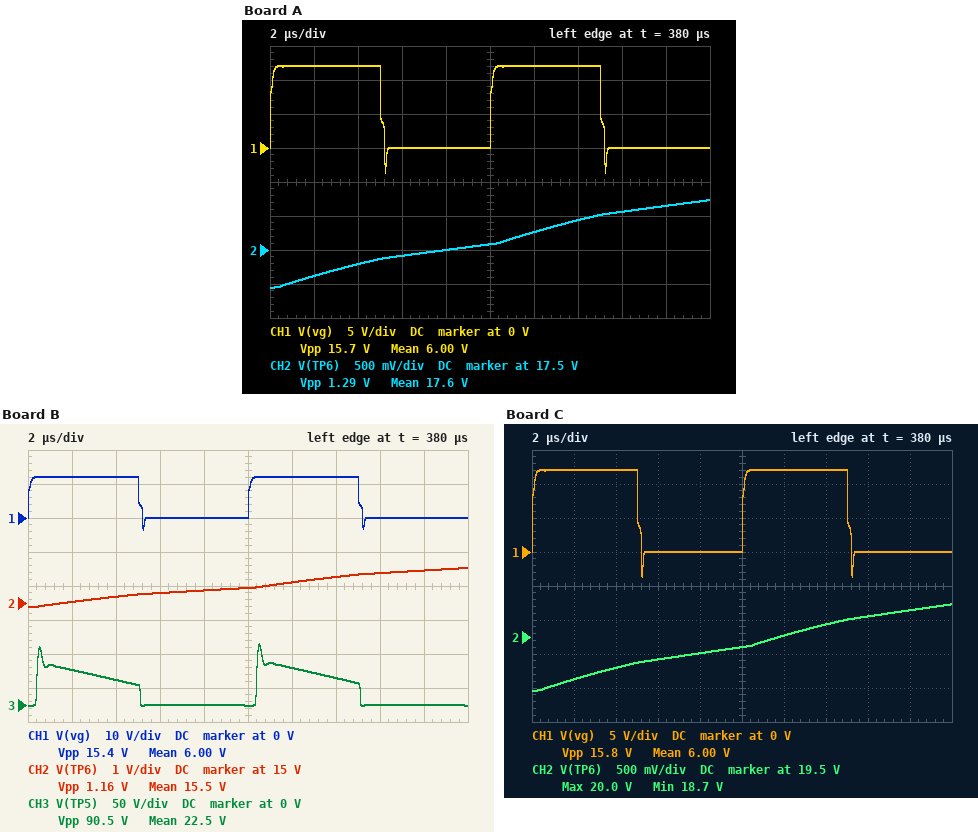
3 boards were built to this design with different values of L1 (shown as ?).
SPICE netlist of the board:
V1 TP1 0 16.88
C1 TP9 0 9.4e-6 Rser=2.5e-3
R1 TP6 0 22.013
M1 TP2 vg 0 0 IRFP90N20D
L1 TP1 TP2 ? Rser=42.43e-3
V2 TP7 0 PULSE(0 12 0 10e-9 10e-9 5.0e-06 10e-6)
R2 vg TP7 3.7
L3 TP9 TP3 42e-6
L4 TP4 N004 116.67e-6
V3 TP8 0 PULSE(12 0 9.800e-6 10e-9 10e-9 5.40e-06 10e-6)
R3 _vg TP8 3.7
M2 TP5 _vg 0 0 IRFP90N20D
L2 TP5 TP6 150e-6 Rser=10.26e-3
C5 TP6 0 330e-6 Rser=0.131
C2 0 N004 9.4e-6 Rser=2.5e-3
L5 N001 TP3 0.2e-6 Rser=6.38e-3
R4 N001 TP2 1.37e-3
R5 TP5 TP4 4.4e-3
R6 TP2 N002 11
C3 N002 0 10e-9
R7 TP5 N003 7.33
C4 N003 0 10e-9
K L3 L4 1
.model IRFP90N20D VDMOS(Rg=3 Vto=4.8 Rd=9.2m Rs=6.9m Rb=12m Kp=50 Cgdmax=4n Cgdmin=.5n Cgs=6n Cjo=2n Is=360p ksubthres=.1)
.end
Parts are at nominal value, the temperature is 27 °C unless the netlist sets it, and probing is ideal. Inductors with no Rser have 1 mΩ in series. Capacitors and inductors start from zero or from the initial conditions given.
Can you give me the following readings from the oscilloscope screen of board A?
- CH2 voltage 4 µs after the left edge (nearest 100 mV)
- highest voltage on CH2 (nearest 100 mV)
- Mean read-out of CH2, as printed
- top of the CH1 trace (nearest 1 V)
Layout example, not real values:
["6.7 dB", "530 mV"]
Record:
["17.3 V", "18.2 V", "17.6 V", "12 V"]
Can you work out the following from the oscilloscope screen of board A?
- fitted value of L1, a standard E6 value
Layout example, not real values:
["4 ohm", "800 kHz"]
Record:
["47 µH"]
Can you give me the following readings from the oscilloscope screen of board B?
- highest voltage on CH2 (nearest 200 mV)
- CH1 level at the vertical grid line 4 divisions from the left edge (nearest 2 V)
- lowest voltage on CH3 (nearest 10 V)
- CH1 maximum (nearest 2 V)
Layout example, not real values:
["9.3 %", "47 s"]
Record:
["16.0 V", "0 V", "0 V", "12 V"]
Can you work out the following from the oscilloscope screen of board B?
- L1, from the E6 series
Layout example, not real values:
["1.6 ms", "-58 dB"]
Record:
["68 µH"]
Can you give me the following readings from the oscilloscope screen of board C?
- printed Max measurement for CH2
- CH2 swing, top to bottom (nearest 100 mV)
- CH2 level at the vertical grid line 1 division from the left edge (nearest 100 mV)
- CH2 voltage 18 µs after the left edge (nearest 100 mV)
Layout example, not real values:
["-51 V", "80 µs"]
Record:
["20.0 V", "1.3 V", "18.9 V", "19.9 V"]
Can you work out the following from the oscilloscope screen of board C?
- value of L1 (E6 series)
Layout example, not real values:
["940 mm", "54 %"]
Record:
["33 µH"]
